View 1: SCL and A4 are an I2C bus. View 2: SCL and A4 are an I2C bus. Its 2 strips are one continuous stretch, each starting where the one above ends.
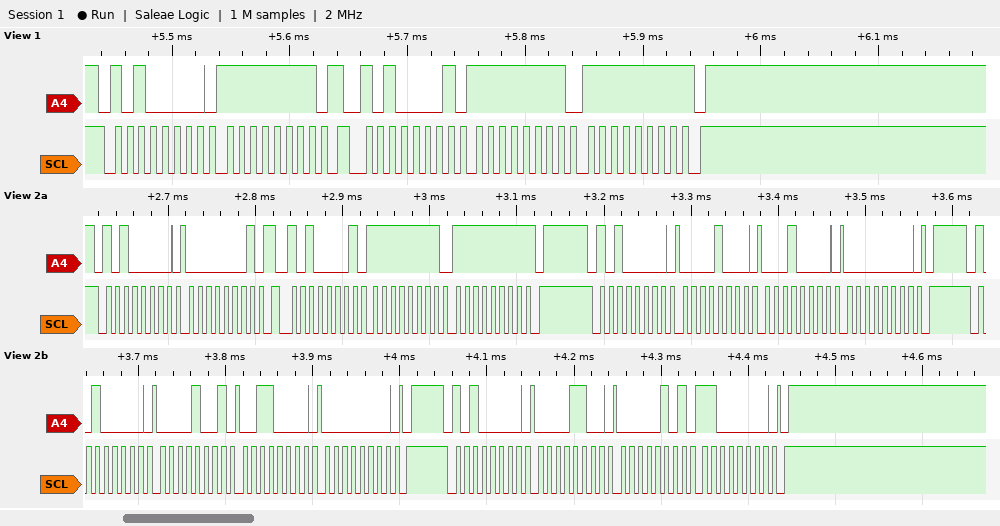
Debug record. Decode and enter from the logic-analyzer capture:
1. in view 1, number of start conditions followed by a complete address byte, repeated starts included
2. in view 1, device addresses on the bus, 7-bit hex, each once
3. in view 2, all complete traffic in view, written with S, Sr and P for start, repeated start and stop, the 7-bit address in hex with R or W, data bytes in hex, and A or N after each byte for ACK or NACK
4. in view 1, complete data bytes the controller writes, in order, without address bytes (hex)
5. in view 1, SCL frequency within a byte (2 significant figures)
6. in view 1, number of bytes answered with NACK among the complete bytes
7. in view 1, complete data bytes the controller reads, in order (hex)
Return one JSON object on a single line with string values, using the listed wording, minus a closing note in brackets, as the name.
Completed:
{"in view 1, number of start conditions followed by a complete address byte, repeated starts included": "2", "in view 1, device addresses on the bus, 7-bit hex, each once": "0x50", "in view 2, all complete traffic in view, written with S, Sr and P for start, repeated start and stop, the 7-bit address in hex with R or W, data bytes in hex, and A or N after each byte for ACK or NACK": "S 50W A 01 A Sr 50R A FF A FF N P S 50W A 08 A 10 A 00 A P S 50W A 09 A 30 A 00 A P S 50W A 0C A 05 A C0 A P", "in view 1, complete data bytes the controller writes, in order, without address bytes": "FF", "in view 1, SCL frequency within a byte": "100 kHz", "in view 1, number of bytes answered with NACK among the complete bytes": "1", "in view 1, complete data bytes the controller reads, in order": "FF FF"}
